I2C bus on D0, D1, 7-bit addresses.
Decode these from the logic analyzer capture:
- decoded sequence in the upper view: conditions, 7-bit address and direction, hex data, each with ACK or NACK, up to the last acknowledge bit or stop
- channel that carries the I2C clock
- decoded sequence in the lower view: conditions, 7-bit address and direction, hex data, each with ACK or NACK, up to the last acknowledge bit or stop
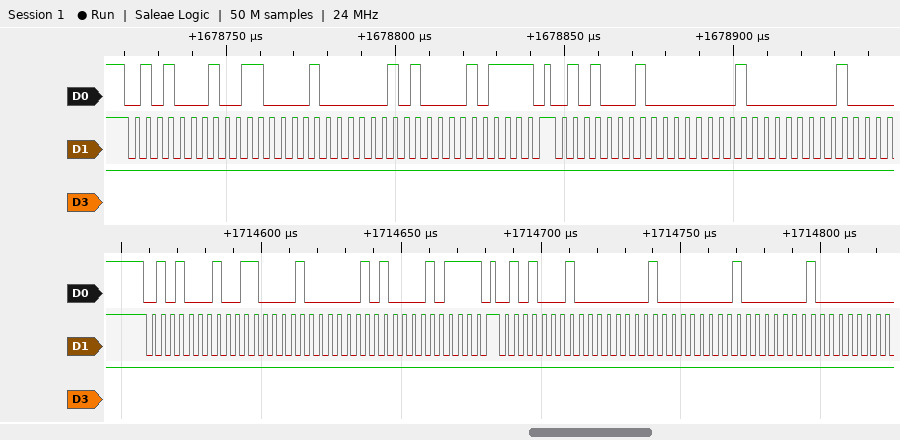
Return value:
start, address 28 read ACK, 61 ACK, 05 ACK, 17 NACK, stop, start, address 28 read ACK, 01 ACK, 01 ACK
D1
start, address 28 read ACK, 61 ACK, 05 ACK, 17 NACK, stop, start, address 28 read ACK, 01 ACK, 01 ACK, 02 ACK
